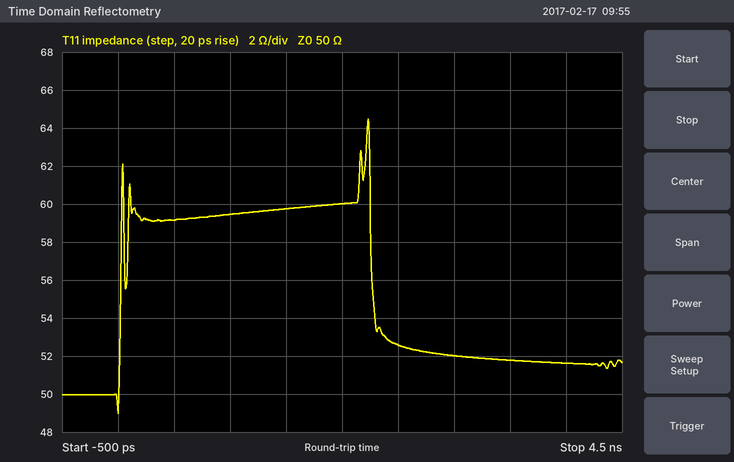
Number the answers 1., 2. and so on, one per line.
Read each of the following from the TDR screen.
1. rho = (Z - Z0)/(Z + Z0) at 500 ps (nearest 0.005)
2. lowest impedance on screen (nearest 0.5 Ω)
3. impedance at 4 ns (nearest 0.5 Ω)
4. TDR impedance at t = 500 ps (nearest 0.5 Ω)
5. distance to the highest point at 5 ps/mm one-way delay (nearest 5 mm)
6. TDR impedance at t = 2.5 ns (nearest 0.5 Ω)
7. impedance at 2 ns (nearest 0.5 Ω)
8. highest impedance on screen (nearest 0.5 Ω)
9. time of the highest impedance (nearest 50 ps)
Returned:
1. +0.085
2. 49.0 Ω
3. 51.5 Ω
4. 59.0 Ω
5. 225 mm
6. 52.5 Ω
7. 60.0 Ω
8. 64.5 Ω
9. 2.25 ns
